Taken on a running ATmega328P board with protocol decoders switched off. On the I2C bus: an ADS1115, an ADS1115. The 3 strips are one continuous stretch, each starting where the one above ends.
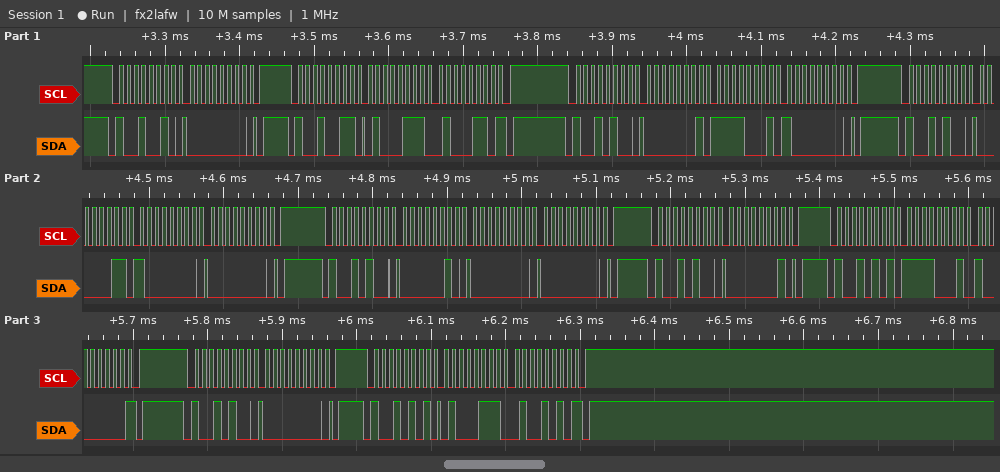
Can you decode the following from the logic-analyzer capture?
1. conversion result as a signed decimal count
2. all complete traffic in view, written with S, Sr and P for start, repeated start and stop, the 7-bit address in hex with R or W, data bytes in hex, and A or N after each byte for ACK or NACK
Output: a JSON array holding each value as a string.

["18246", "S 49W A 00 A P S 49R A 47 A 46 N P S 4AW A 01 A F1 A 80 A P S 4AW A 03 A 80 A 00 A P S 4AW A 02 A 00 A 00 A P S 4AW A 01 A P S 4AR A F1 A 80 N P S 4AW A 00 A P S 4AR A 47 A 4A N P"]
